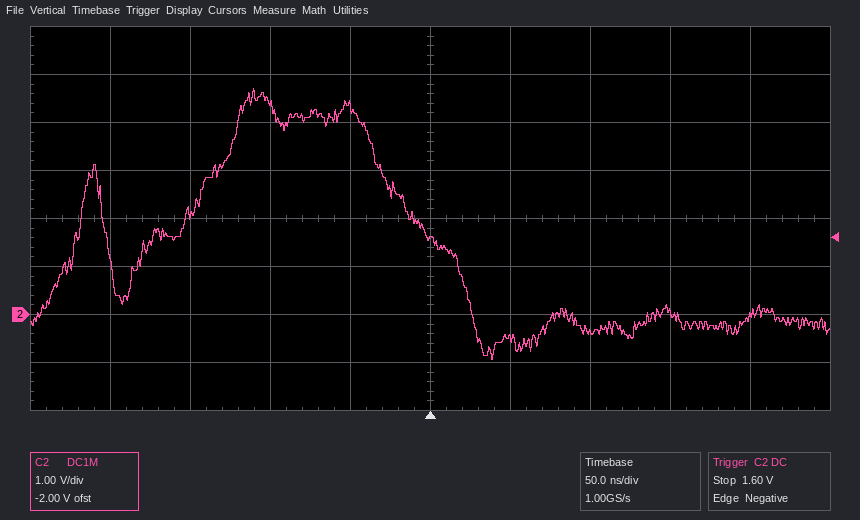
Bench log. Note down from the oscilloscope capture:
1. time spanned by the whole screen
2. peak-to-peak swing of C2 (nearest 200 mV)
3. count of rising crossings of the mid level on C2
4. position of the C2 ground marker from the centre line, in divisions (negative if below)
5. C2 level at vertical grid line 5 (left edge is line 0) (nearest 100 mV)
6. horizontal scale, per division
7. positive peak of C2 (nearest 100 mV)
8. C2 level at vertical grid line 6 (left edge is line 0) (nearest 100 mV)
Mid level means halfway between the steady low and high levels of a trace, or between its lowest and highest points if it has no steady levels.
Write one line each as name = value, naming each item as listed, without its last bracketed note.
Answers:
time spanned by the whole screen = 500 ns
peak-to-peak swing of C2 = 5.6 V
count of rising crossings of the mid level on C2 = 2
position of the C2 ground marker from the centre line, in divisions = -2.0 div
C2 level at vertical grid line 5 (left edge is line 0) = 1.6 V
horizontal scale, per division = 50 ns
positive peak of C2 = 4.7 V
C2 level at vertical grid line 6 (left edge is line 0) = -500 mV
